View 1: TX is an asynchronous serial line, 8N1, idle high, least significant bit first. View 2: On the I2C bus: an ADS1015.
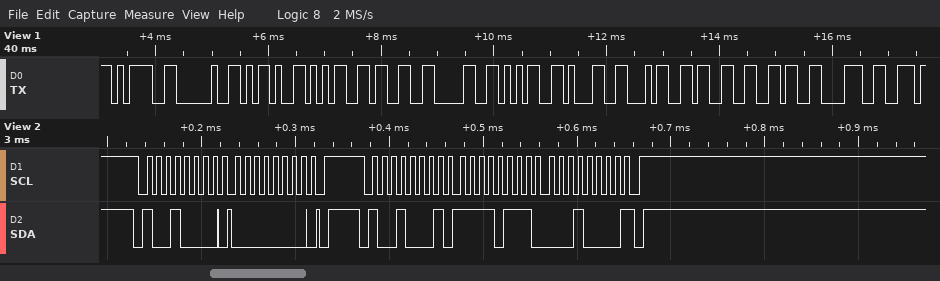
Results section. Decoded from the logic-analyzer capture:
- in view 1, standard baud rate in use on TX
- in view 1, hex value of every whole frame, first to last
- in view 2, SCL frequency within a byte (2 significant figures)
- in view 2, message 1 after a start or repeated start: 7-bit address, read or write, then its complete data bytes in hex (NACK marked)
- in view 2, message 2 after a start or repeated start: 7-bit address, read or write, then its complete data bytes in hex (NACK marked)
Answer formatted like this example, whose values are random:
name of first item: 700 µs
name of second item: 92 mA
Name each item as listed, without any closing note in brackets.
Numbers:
in view 1, standard baud rate in use on TX: 9600 baud
in view 1, hex value of every whole frame, first to last: 3D 20 2D 35 33 30 35 31 34 33 36 38
in view 2, SCL frequency within a byte: 100 kHz
in view 2, message 1 after a start or repeated start: 7-bit address, read or write, then its complete data bytes in hex: 0x48 write: 00
in view 2, message 2 after a start or repeated start: 7-bit address, read or write, then its complete data bytes in hex: 0x48 read: F7 10 NACK
